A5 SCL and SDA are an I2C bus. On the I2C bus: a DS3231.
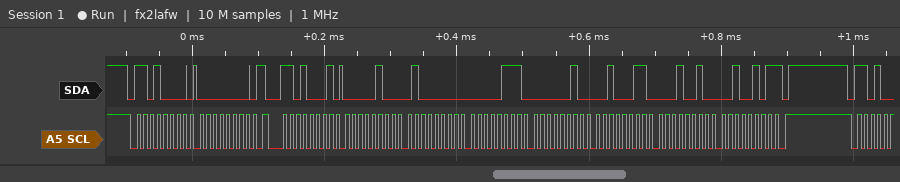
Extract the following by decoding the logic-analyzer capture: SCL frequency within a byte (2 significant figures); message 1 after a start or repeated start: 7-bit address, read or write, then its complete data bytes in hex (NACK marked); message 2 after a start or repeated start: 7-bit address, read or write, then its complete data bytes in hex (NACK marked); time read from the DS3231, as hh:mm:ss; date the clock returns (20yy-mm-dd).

100 kHz
0x68 write: 00
0x68 read: 04 40 07 02 23 12 25 NACK
07:40:04
2025-12-23
